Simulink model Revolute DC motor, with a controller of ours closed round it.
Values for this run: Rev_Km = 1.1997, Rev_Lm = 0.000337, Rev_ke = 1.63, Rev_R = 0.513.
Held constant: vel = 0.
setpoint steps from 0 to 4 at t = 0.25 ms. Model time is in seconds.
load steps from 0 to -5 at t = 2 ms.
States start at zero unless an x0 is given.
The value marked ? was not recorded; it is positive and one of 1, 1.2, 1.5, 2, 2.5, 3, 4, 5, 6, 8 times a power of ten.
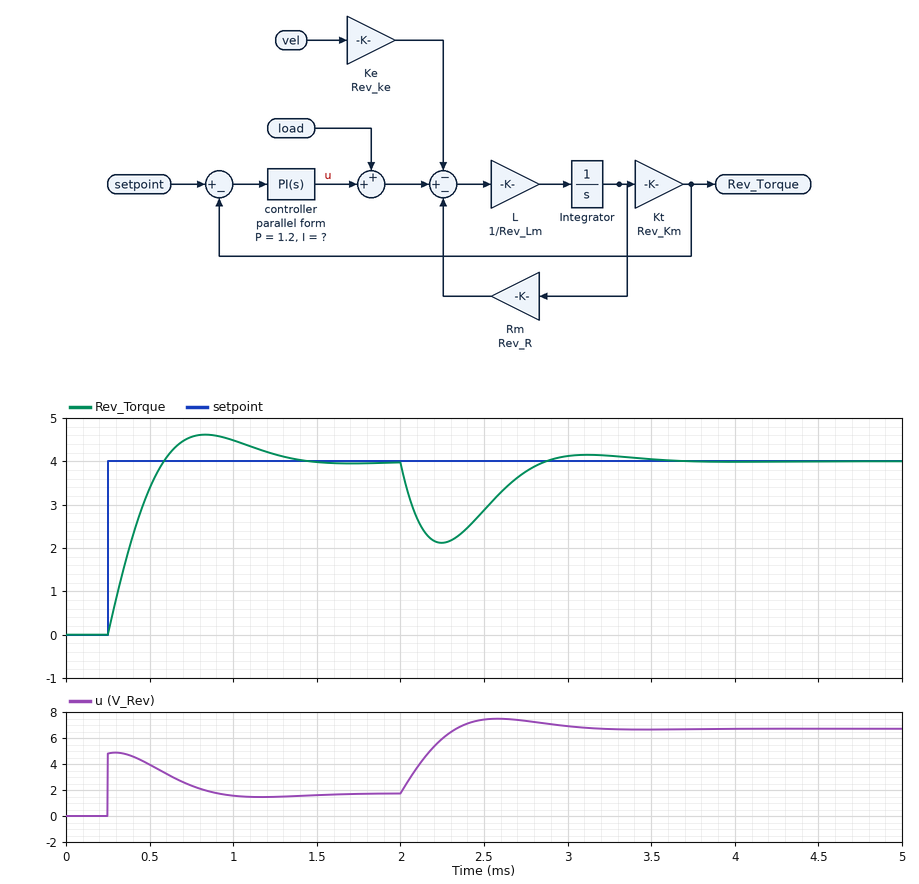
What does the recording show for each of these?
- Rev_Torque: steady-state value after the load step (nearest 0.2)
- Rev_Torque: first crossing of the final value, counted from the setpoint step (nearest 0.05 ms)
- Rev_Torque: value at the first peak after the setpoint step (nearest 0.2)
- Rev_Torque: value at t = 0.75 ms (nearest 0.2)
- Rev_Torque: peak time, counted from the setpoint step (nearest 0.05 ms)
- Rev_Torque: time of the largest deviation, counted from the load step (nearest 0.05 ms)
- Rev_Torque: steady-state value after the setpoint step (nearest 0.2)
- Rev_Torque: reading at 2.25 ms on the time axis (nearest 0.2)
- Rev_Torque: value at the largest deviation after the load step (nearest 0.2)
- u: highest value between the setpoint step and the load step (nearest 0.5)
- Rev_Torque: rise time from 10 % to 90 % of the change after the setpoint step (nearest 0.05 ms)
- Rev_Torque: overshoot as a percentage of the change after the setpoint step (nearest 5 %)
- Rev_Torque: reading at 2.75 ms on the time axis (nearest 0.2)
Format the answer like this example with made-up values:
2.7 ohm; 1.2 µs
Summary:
4.0; 0.35 ms; 4.6; 4.6; 0.60 ms; 0.25 ms; 4.0; 2.2; 2.2; 5.0; 0.25 ms; 15 %; 3.8
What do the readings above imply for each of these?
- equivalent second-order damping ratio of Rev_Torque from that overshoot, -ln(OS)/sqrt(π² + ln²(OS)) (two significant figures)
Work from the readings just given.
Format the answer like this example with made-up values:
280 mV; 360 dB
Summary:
0.52
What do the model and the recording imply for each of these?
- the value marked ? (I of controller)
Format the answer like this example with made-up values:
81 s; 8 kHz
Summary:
6000
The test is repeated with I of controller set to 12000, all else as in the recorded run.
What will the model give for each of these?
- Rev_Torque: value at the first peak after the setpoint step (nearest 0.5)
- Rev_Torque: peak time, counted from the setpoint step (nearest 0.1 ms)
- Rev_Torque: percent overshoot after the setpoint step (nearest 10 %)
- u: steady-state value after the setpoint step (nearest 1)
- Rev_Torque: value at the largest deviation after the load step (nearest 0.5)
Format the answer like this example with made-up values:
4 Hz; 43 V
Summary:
5.0; 0.4 ms; 30 %; 2; 2.5
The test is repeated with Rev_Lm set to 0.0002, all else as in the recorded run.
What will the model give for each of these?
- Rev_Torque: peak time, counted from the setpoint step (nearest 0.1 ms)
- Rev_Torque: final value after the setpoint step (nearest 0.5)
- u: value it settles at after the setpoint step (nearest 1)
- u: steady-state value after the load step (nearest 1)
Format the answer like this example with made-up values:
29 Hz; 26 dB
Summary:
0.5 ms; 4.0; 2; 7
